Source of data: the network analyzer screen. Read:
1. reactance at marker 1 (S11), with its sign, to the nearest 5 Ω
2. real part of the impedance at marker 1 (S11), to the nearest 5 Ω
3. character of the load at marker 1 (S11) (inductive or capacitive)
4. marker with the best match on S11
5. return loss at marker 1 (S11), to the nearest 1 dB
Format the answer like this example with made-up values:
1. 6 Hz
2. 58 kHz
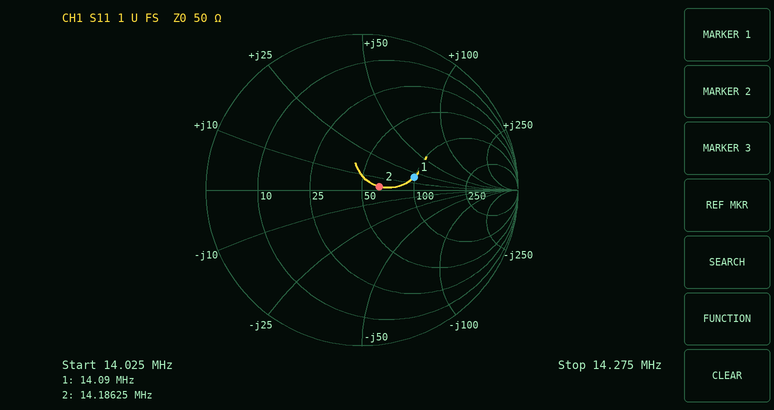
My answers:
1. +20 Ω
2. 100 Ω
3. inductive
4. marker 2
5. 9 dB
